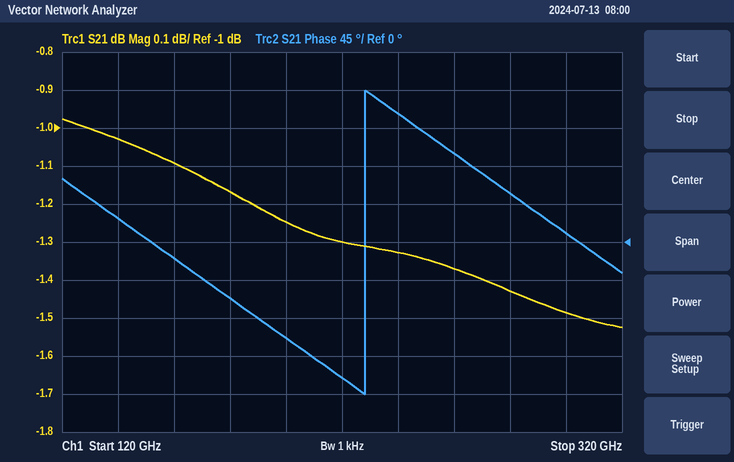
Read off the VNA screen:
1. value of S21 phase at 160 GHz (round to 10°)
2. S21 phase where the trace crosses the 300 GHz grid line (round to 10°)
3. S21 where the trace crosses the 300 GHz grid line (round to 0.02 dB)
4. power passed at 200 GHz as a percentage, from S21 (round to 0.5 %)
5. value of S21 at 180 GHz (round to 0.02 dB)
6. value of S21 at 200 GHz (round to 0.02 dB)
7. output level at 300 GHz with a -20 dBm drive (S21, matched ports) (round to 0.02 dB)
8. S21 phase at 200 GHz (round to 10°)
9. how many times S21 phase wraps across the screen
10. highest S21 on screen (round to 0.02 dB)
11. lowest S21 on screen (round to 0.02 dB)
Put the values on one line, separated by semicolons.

-20°; 10°; -1.48 dB; 75.0 %; -1.16 dB; -1.24 dB; -21.48 dBm; -110°; 1; -0.98 dB; -1.52 dB
